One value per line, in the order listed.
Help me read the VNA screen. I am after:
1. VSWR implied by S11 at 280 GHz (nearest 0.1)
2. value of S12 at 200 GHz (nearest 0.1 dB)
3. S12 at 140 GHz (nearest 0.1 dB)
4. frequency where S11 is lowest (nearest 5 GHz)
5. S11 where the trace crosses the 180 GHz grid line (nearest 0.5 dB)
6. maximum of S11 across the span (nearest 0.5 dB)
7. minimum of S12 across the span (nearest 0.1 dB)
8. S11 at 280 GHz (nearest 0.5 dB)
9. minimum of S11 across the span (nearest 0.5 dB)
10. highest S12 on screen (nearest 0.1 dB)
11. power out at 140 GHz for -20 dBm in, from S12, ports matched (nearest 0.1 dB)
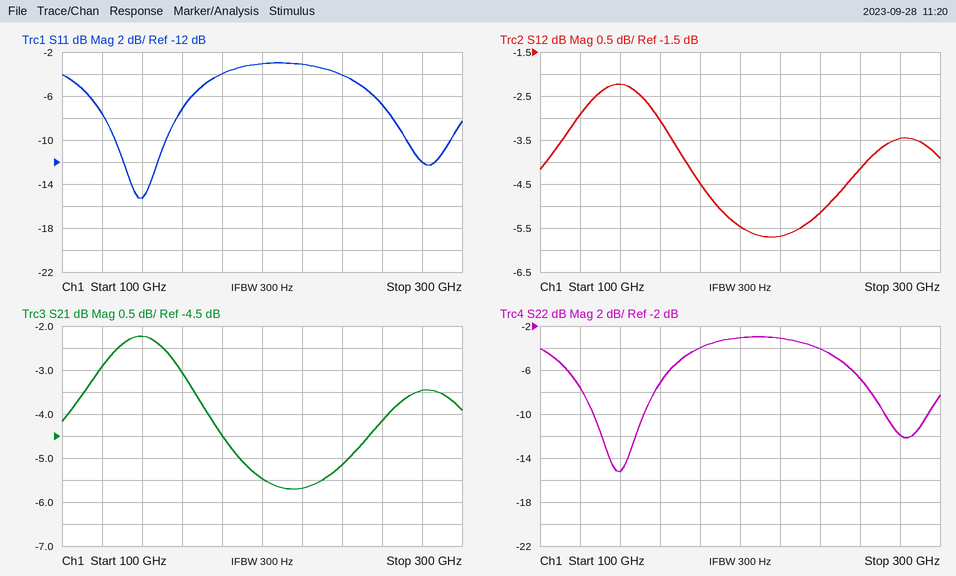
1.7
-5.5 dB
-2.2 dB
140 GHz
-4.0 dB
-3.0 dB
-5.7 dB
-12.0 dB
-15.5 dB
-2.2 dB
-22.2 dBm
